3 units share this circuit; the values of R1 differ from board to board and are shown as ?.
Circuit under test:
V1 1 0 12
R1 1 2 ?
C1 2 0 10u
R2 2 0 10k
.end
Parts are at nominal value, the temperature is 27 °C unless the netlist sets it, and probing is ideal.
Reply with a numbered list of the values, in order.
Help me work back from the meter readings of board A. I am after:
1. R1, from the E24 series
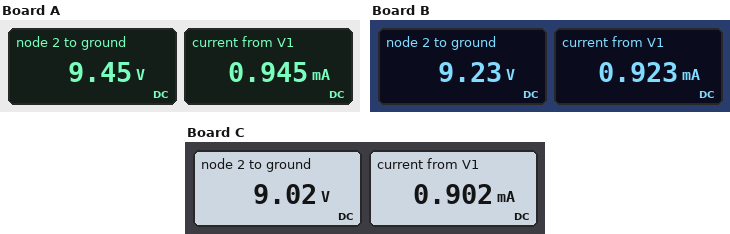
1. 2.7 kΩ
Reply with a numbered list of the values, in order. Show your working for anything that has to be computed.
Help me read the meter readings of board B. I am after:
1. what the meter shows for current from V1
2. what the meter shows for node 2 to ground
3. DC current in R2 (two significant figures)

1. 0.923 mA
2. 9.23 V
3. (9.23 V) / 10 kΩ = 920 µA
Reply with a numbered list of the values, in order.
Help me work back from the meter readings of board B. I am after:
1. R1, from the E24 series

1. 3 kΩ
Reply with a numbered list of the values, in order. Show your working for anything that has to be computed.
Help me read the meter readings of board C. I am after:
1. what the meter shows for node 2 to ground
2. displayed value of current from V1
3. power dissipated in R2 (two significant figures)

1. 9.02 V
2. 0.902 mA
3. (9.02 V)^2 / 10 kΩ = 8.1 mW
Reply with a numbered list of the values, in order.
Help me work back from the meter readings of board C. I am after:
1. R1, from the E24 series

1. 3.3 kΩ
